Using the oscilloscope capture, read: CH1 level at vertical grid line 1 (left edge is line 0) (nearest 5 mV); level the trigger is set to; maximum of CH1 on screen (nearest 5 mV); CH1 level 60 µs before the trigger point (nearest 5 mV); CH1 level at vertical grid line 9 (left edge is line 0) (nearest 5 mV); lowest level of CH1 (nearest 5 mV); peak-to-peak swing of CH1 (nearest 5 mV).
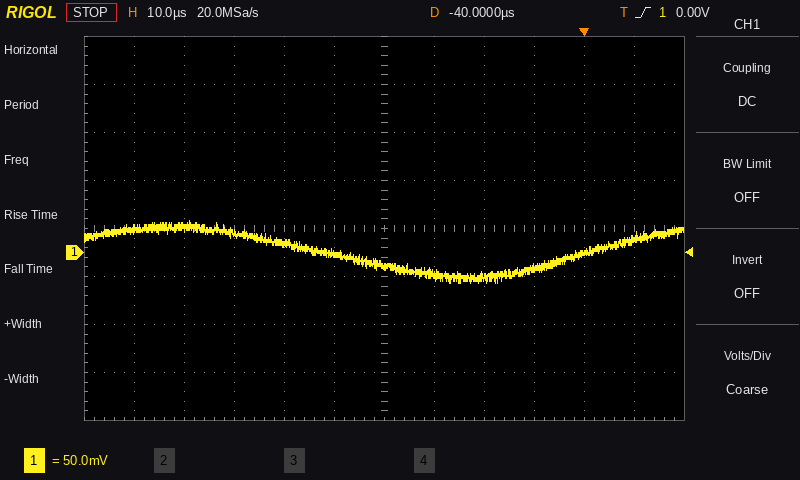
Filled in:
25 mV
0.00 V
35 mV
10 mV
-15 mV
-30 mV
65 mV
